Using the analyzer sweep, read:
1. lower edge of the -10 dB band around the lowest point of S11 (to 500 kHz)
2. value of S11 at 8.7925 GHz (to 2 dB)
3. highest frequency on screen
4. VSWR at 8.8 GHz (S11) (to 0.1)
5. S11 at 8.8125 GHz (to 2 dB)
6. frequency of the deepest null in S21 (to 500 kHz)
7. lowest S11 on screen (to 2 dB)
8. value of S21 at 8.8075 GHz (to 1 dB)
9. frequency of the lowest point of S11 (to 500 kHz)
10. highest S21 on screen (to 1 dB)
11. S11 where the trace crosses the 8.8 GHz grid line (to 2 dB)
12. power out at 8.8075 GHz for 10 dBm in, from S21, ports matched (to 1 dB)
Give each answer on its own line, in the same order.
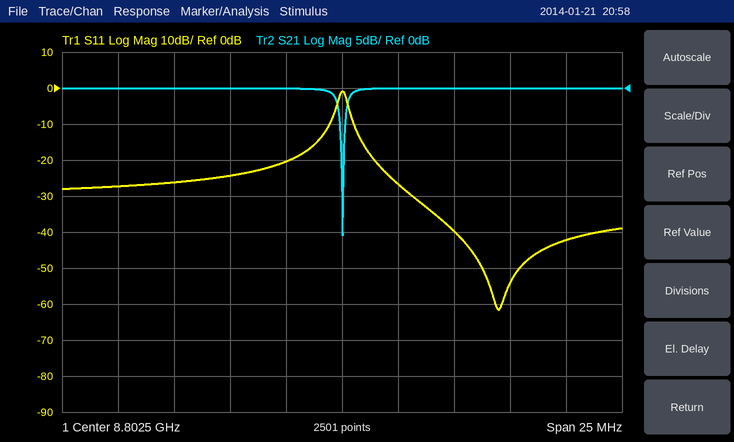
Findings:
8.8030 GHz
-28 dB
8.815 GHz
1.2
-42 dB
8.8025 GHz
-62 dB
0 dB
8.8095 GHz
0 dB
-20 dB
10 dBm
